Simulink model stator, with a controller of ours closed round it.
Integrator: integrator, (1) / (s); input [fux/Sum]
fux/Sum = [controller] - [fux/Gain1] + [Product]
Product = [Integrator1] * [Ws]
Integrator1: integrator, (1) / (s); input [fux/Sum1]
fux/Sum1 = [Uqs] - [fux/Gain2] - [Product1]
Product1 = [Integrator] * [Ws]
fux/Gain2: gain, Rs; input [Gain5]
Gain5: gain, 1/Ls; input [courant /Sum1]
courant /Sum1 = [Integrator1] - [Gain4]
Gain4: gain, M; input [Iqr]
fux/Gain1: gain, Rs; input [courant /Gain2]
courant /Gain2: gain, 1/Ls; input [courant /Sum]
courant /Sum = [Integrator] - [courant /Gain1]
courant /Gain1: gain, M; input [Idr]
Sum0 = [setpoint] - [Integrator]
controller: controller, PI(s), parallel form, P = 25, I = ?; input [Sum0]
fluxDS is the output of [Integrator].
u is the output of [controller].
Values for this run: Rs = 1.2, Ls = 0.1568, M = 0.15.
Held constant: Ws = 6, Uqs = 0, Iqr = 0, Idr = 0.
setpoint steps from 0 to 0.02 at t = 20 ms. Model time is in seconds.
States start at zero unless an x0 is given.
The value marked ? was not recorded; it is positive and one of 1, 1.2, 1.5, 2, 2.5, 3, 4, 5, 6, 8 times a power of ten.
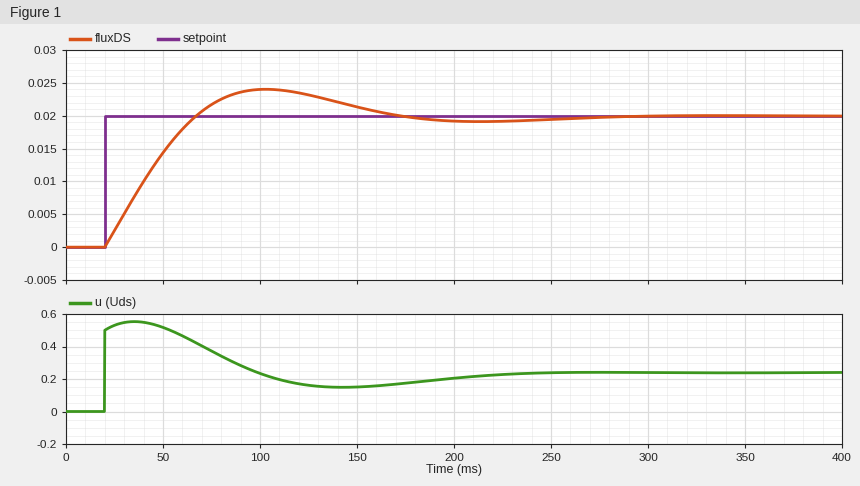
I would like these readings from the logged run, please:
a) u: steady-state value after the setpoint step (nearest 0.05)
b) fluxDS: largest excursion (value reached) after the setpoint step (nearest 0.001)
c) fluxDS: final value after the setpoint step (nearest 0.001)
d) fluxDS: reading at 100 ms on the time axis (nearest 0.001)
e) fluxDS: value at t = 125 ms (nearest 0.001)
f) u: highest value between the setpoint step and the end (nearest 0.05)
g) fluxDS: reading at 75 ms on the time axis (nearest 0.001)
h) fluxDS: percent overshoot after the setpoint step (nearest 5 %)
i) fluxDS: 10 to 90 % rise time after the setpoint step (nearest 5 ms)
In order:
0.25
0.024
0.020
0.024
0.023
0.55
0.022
20 %
35 ms
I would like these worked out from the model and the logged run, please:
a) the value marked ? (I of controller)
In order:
1000
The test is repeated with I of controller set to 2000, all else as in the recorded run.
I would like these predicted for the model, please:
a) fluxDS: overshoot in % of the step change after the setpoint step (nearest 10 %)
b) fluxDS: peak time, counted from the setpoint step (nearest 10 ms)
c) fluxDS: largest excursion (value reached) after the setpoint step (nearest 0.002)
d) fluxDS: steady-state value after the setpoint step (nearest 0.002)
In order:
30 %
60 ms
0.026
0.020
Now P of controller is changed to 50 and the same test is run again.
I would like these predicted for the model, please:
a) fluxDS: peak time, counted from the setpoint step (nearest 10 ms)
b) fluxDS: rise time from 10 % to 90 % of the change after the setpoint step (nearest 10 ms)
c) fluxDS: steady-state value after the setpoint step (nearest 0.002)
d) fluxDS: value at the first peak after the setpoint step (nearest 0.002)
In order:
70 ms
30 ms
0.020
0.022
